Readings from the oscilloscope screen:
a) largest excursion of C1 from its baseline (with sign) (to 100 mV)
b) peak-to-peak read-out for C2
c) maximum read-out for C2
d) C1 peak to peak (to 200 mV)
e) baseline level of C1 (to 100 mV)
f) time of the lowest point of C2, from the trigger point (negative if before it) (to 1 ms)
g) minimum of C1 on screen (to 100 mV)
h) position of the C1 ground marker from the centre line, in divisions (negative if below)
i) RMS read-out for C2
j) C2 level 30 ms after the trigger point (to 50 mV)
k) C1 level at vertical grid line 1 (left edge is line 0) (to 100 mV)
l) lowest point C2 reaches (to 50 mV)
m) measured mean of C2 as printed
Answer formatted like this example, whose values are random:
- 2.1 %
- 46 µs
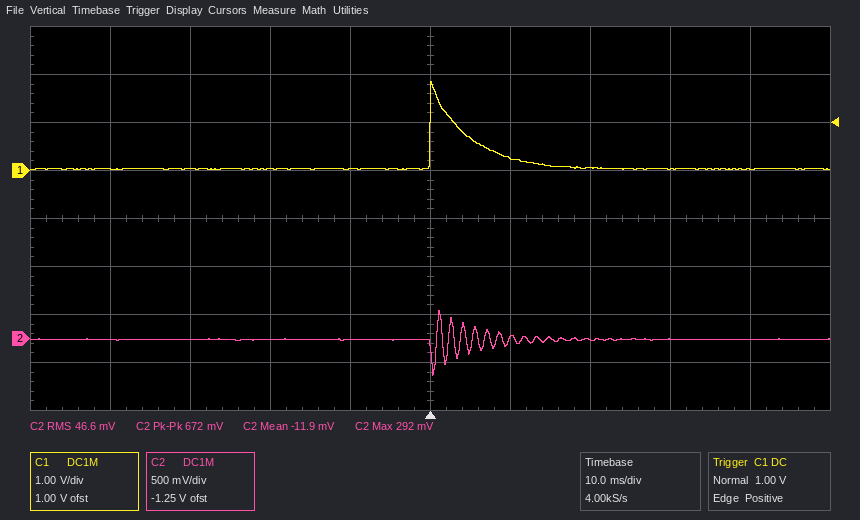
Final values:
- +1.8 V
- 672 mV
- 292 mV
- 1.8 V
- 0.0 V
- 0 ms
- 0.0 V
- +1.0 div
- 46.6 mV
- 0 mV
- 0.0 V
- -400 mV
- -11.9 mV
